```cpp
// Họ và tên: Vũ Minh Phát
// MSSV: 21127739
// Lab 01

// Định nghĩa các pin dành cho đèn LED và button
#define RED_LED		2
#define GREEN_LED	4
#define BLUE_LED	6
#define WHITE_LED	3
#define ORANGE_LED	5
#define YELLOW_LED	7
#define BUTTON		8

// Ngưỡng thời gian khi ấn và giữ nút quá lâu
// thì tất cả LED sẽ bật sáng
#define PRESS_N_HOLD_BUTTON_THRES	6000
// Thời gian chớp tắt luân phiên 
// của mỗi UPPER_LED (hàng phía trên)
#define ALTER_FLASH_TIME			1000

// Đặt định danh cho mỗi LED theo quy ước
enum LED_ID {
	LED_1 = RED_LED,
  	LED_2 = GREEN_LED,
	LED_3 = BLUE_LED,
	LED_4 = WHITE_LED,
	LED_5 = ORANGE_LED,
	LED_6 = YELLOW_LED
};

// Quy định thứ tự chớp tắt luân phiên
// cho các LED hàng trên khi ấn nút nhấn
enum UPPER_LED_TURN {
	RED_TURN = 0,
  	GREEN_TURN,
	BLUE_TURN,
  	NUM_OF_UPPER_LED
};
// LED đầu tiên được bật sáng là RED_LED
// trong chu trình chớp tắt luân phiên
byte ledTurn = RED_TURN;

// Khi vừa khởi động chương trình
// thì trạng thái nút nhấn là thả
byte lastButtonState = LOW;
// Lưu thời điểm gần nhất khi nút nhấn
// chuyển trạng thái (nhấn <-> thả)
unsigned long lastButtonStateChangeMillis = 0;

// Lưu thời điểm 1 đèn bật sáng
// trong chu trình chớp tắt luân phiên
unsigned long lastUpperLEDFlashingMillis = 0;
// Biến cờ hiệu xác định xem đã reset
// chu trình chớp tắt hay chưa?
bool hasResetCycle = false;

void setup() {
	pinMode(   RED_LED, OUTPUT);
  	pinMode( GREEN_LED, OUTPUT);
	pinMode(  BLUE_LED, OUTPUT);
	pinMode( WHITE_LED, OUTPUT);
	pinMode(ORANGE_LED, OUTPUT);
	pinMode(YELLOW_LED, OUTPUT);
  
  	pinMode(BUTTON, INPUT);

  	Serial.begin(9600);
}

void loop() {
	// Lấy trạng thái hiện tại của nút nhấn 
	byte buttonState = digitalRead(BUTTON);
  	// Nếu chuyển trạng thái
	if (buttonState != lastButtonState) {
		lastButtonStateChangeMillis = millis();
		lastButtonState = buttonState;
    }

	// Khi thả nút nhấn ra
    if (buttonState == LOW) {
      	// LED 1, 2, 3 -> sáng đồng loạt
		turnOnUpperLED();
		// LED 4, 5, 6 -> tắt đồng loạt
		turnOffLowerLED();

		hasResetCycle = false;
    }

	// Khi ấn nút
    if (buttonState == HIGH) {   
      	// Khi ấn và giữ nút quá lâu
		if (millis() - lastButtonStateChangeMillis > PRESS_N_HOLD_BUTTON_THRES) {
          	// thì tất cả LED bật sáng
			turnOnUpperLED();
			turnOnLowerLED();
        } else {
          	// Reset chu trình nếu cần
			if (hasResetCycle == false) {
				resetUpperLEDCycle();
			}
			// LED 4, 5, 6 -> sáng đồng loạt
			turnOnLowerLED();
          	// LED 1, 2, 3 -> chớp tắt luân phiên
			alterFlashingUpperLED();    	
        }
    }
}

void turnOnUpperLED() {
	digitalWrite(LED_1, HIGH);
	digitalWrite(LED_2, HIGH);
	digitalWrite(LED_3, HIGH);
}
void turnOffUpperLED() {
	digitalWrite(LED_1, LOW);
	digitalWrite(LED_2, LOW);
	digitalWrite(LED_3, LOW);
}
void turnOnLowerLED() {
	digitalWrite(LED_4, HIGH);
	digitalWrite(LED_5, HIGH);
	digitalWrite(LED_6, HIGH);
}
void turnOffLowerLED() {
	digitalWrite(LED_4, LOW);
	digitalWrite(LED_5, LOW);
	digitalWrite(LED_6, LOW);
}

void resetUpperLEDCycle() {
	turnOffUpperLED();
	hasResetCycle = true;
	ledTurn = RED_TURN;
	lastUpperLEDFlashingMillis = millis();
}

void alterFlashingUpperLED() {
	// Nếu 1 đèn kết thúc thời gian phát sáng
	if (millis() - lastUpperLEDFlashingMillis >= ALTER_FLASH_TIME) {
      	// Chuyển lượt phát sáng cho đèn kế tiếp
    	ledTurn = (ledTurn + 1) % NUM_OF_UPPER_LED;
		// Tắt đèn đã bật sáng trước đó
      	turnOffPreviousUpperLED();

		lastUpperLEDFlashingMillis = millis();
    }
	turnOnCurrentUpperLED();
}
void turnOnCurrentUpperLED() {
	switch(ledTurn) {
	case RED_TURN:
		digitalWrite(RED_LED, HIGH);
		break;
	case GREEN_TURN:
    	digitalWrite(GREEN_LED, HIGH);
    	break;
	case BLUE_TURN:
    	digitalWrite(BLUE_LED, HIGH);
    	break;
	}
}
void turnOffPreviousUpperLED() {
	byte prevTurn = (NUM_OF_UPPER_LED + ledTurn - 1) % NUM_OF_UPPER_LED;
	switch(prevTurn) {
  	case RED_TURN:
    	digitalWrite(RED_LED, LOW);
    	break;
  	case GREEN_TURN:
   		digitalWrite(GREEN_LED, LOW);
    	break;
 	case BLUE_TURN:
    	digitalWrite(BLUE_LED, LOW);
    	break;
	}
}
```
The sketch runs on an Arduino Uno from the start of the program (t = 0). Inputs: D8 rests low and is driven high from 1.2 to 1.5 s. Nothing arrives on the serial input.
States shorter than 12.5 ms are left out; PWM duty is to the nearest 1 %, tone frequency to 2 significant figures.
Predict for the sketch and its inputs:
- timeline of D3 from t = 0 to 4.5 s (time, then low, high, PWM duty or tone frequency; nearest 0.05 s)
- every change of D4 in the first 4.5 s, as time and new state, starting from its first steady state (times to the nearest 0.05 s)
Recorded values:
0 s low; 1.2 s high; 1.5 s low
0 s high; 1.2 s low; 1.5 s high
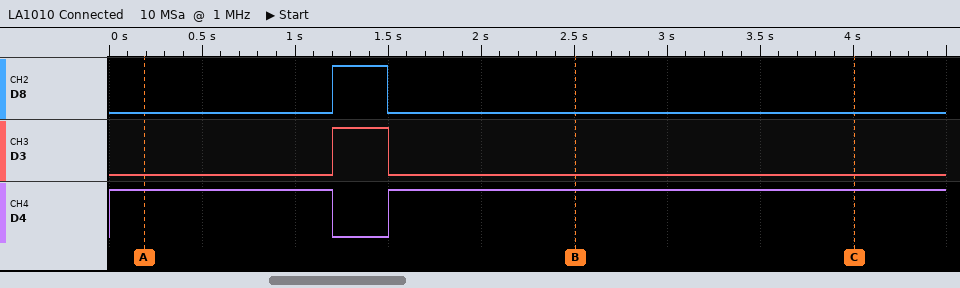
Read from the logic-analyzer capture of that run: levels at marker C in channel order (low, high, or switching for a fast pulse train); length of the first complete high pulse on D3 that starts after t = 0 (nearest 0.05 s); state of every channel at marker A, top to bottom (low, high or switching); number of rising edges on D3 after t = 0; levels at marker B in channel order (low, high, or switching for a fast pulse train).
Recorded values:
D8 low, D3 low, D4 high
0.30 s
D8 low, D3 low, D4 high
1
D8 low, D3 low, D4 high
